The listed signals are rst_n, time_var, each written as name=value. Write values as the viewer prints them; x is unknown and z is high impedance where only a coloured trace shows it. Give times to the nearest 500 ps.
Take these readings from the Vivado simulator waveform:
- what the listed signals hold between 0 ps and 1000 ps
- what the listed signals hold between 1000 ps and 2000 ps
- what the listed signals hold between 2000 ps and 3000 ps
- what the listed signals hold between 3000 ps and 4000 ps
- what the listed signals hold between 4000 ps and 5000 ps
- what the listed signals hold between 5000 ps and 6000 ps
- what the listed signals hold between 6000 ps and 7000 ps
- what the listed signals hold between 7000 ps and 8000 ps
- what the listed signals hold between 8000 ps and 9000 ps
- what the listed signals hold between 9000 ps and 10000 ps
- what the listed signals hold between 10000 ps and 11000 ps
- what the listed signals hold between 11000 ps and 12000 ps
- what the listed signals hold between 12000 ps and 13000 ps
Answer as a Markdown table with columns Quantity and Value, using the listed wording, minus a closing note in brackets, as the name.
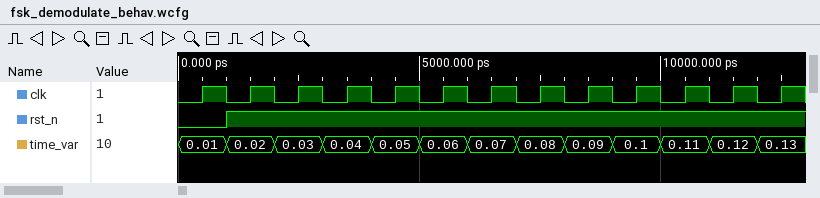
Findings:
| Quantity | Value |
|---|---|
| what the listed signals hold between 0 ps and 1000 ps | rst_n=0, time_var=0.01 |
| what the listed signals hold between 1000 ps and 2000 ps | rst_n=1, time_var=0.02 |
| what the listed signals hold between 2000 ps and 3000 ps | rst_n=1, time_var=0.03 |
| what the listed signals hold between 3000 ps and 4000 ps | rst_n=1, time_var=0.04 |
| what the listed signals hold between 4000 ps and 5000 ps | rst_n=1, time_var=0.05 |
| what the listed signals hold between 5000 ps and 6000 ps | rst_n=1, time_var=0.06 |
| what the listed signals hold between 6000 ps and 7000 ps | rst_n=1, time_var=0.07 |
| what the listed signals hold between 7000 ps and 8000 ps | rst_n=1, time_var=0.08 |
| what the listed signals hold between 8000 ps and 9000 ps | rst_n=1, time_var=0.09 |
| what the listed signals hold between 9000 ps and 10000 ps | rst_n=1, time_var=0.1 |
| what the listed signals hold between 10000 ps and 11000 ps | rst_n=1, time_var=0.11 |
| what the listed signals hold between 11000 ps and 12000 ps | rst_n=1, time_var=0.12 |
| what the listed signals hold between 12000 ps and 13000 ps | rst_n=1, time_var=0.13 |
